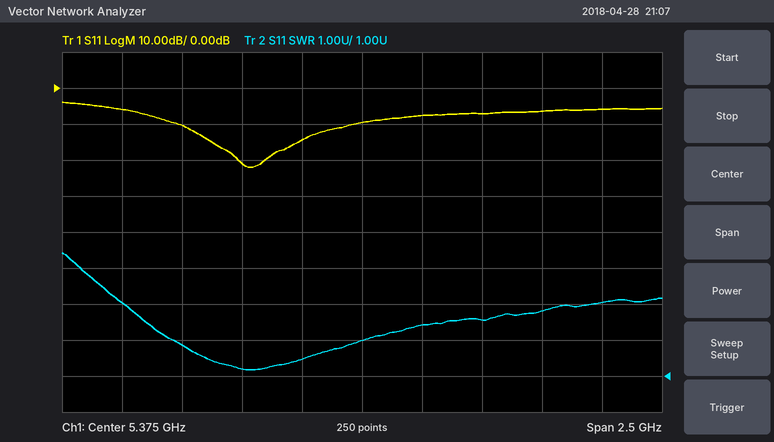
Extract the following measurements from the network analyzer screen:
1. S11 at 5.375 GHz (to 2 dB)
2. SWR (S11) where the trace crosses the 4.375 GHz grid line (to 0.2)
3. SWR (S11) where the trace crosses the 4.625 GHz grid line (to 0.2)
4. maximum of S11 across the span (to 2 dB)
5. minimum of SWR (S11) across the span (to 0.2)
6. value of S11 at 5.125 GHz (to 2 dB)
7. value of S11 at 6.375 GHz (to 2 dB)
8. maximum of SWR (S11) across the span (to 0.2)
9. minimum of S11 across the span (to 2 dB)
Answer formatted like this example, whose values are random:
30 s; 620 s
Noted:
-10 dB; 3.0; 1.8; -4 dB; 1.2; -14 dB; -6 dB; 4.4; -22 dB
